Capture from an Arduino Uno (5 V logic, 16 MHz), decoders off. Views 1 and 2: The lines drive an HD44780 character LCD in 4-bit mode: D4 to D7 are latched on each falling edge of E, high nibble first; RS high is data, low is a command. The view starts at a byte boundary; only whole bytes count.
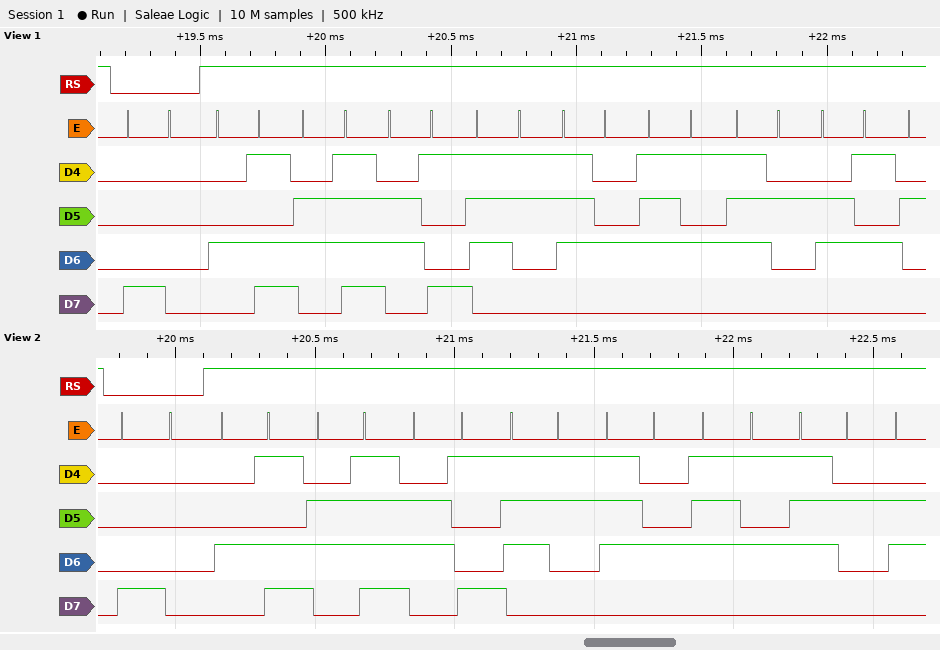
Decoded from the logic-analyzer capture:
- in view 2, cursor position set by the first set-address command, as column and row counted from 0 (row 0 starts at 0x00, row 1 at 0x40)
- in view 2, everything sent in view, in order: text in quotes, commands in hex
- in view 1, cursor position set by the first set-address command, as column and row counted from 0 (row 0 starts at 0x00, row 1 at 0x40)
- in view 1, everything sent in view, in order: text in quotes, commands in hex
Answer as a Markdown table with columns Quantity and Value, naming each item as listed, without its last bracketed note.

| Quantity | Value |
|---|---|
| in view 2, cursor position set by the first set-address command, as column and row counted from 0 | column 0, row 0 |
| in view 2, everything sent in view, in order: text in quotes, commands in hex | 0x80 "Moistur" |
| in view 1, cursor position set by the first set-address command, as column and row counted from 0 | column 0, row 0 |
| in view 1, everything sent in view, in order: text in quotes, commands in hex | 0x80 "Moisture" |
